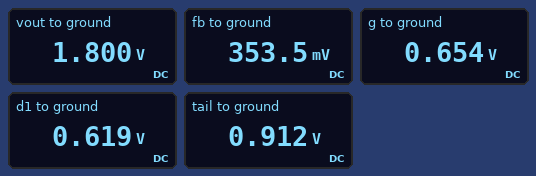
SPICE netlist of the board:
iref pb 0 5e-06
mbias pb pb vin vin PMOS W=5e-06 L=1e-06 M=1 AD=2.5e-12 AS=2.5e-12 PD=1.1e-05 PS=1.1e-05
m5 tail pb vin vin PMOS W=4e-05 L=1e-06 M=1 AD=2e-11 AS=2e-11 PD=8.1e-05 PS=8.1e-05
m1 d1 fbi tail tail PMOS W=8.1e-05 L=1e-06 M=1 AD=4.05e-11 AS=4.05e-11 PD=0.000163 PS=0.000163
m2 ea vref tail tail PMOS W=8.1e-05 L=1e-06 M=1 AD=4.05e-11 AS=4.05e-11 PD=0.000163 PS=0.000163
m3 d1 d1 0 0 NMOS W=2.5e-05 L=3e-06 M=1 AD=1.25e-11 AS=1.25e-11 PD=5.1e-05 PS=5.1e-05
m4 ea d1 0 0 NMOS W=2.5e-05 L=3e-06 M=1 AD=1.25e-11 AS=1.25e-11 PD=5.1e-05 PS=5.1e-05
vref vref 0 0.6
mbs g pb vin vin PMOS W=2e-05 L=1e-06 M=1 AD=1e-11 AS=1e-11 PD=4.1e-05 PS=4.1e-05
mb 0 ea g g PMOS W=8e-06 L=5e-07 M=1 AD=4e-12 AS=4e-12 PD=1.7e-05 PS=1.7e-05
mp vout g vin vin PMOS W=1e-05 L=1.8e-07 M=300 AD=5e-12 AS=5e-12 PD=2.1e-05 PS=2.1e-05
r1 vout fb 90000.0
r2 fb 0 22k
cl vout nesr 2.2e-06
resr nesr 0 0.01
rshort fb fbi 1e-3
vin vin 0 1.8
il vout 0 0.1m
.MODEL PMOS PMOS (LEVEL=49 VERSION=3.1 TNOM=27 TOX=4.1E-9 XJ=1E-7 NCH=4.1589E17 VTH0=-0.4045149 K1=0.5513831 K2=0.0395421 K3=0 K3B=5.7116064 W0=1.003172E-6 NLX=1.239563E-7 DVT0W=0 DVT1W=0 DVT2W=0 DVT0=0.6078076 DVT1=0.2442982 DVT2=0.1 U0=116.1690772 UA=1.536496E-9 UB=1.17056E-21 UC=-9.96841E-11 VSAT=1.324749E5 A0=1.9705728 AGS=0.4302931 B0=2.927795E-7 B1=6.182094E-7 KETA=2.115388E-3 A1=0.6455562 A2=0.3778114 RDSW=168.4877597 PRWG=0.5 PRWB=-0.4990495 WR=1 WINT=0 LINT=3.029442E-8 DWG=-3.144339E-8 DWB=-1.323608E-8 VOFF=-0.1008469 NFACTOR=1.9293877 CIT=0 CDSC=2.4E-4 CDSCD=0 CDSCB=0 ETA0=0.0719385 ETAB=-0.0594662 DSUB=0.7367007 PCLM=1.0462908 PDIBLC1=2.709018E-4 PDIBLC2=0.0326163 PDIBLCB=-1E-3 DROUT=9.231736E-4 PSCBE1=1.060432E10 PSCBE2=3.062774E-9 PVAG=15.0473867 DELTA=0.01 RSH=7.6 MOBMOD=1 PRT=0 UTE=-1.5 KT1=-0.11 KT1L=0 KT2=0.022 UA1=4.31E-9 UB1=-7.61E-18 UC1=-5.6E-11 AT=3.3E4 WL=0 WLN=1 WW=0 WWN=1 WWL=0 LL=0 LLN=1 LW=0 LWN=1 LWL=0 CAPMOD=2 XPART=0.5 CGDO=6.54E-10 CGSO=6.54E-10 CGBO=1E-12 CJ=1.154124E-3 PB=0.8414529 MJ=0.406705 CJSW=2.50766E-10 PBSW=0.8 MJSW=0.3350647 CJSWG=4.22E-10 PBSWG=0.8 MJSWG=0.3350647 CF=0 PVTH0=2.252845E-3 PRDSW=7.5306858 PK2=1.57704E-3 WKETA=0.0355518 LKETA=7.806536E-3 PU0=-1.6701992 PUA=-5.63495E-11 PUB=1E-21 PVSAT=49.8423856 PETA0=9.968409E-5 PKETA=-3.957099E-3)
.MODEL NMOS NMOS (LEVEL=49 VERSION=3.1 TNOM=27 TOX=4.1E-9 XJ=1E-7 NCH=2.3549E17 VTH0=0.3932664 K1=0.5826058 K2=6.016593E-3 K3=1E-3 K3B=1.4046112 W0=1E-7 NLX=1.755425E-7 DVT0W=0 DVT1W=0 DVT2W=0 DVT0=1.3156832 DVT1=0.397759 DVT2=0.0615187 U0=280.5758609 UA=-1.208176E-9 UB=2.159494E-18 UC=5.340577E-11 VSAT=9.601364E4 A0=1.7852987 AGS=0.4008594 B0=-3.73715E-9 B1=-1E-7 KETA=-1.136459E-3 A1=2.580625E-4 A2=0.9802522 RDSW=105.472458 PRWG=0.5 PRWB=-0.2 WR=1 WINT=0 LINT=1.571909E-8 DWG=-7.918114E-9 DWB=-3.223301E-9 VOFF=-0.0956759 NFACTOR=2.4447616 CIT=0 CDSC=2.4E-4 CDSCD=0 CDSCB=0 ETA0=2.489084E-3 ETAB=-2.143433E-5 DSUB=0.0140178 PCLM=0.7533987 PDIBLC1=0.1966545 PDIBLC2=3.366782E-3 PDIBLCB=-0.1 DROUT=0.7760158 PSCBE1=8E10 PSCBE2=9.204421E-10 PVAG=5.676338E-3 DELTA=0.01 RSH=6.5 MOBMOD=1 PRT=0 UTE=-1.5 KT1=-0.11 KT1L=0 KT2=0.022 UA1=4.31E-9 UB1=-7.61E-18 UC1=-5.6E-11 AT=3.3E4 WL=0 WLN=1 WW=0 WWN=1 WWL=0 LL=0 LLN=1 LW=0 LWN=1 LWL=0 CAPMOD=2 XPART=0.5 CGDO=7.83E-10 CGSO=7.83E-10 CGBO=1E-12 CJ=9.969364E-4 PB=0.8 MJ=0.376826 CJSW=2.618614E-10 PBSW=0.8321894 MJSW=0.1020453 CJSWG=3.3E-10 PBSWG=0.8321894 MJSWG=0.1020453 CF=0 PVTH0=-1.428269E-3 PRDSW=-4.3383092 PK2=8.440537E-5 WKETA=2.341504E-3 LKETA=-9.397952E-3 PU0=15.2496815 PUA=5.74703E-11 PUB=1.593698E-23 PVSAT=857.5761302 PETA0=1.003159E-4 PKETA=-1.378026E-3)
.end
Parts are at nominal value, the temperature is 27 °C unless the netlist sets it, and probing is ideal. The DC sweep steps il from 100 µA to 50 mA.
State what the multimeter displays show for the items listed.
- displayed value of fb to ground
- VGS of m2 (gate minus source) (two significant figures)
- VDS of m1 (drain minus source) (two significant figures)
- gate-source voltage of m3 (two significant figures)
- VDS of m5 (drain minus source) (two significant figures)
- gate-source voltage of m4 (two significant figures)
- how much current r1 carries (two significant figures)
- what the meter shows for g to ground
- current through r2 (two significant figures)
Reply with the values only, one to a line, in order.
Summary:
353.5 mV
-310 mV
-290 mV
620 mV
-890 mV
620 mV
16 µA
0.654 V
16 µA
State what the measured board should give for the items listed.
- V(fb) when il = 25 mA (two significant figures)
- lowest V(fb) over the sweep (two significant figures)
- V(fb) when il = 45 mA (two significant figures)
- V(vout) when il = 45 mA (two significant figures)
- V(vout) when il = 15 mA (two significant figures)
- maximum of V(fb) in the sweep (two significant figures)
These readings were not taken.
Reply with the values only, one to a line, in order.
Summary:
350 mV
340 mV
340 mV
1.7 V
1.8 V
350 mV
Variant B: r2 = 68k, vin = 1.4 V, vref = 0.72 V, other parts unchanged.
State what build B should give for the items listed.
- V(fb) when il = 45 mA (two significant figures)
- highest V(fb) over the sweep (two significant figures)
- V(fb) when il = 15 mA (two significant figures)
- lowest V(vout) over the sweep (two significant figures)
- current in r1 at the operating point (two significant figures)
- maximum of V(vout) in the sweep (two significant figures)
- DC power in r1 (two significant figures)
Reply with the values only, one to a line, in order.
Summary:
330 mV
600 mV
580 mV
350 mV
8.9 µA
1.4 V
7.1 µW
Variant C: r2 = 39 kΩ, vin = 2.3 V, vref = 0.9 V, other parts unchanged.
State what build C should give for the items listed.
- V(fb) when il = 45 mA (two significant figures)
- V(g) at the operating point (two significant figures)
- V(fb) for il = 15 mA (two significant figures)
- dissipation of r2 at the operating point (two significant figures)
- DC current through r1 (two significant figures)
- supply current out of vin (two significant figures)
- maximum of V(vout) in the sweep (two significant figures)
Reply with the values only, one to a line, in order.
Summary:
680 mV
660 mV
690 mV
12 µW
18 µA
190 µA
2.3 V
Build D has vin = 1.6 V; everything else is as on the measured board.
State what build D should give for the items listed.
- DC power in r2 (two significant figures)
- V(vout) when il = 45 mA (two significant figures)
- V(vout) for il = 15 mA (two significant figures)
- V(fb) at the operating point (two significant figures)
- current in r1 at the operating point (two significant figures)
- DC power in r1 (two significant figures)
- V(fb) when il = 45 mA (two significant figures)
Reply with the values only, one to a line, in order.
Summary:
4.5 µW
1.5 V
1.6 V
310 mV
14 µA
18 µW
300 mV
